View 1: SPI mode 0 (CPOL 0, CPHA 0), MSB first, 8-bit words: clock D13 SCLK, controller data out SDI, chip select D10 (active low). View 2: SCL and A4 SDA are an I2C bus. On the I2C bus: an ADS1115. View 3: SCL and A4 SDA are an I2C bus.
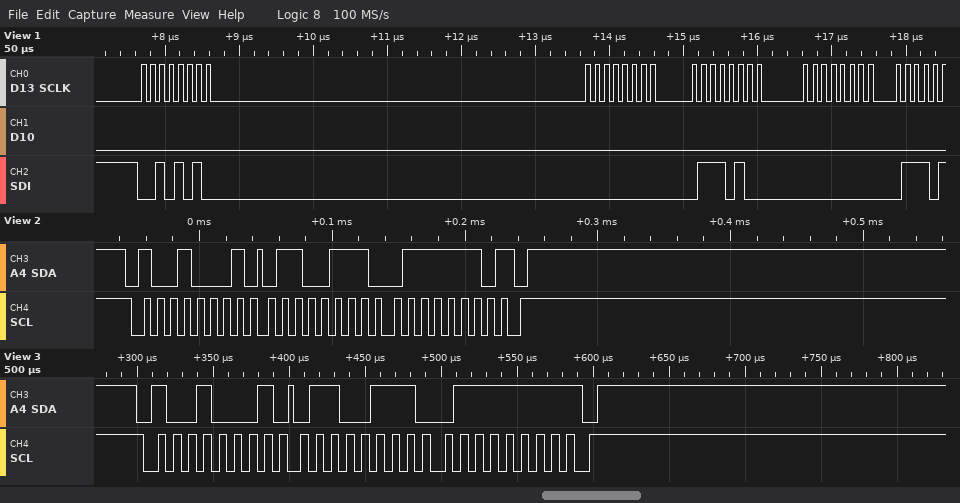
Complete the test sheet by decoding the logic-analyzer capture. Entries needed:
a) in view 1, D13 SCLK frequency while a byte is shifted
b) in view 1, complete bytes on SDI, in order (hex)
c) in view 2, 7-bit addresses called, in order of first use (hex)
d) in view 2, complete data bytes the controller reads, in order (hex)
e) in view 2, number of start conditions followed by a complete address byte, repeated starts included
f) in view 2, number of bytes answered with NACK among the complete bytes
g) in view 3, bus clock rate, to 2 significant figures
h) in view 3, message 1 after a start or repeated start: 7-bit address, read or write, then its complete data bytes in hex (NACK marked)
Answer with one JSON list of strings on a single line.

["8 MHz", "2A 00 74 00", "0x48", "67 7E", "1", "1", "100 kHz", "0x48 read: 67 7F NACK"]
